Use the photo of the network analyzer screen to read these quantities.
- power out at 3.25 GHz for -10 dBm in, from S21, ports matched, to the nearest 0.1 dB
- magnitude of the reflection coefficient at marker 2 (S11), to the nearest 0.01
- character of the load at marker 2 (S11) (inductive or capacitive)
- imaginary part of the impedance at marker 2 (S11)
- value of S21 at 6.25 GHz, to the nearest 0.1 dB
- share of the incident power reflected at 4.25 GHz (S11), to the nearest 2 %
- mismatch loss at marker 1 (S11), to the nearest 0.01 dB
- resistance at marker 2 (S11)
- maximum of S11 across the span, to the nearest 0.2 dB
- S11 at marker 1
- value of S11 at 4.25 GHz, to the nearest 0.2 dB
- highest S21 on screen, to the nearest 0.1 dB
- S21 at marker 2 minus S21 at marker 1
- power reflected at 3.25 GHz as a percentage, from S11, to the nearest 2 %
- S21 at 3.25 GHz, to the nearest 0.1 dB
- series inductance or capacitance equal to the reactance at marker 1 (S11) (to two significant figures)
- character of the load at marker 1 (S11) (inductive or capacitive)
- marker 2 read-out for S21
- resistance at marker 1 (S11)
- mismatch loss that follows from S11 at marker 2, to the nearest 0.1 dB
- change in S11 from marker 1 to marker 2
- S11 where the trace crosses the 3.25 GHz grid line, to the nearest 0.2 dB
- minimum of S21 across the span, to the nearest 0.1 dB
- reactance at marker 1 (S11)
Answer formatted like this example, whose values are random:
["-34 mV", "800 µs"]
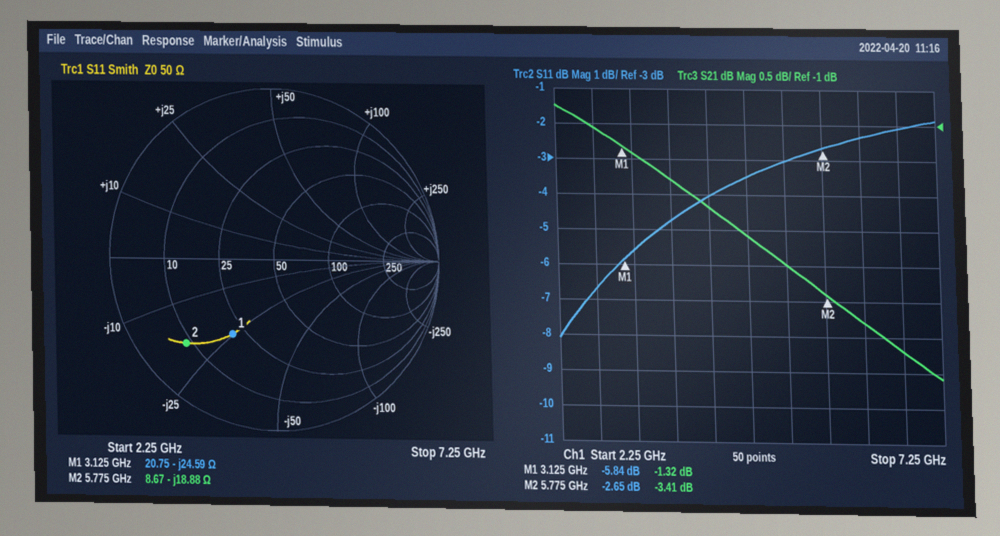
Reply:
["-11.4 dBm", "0.74", "capacitive", "-18.88 Ω", "-3.8 dB", "40 %", "1.31 dB", "8.67 Ω", "-1.8 dB", "-5.84 dB", "-4.0 dB", "-0.7 dB", "-2.09 dB", "28 %", "-1.4 dB", "2.1 pF", "capacitive", "-3.41 dB", "20.75 Ω", "3.4 dB", "3.19 dB", "-5.6 dB", "-4.6 dB", "-24.59 Ω"]
